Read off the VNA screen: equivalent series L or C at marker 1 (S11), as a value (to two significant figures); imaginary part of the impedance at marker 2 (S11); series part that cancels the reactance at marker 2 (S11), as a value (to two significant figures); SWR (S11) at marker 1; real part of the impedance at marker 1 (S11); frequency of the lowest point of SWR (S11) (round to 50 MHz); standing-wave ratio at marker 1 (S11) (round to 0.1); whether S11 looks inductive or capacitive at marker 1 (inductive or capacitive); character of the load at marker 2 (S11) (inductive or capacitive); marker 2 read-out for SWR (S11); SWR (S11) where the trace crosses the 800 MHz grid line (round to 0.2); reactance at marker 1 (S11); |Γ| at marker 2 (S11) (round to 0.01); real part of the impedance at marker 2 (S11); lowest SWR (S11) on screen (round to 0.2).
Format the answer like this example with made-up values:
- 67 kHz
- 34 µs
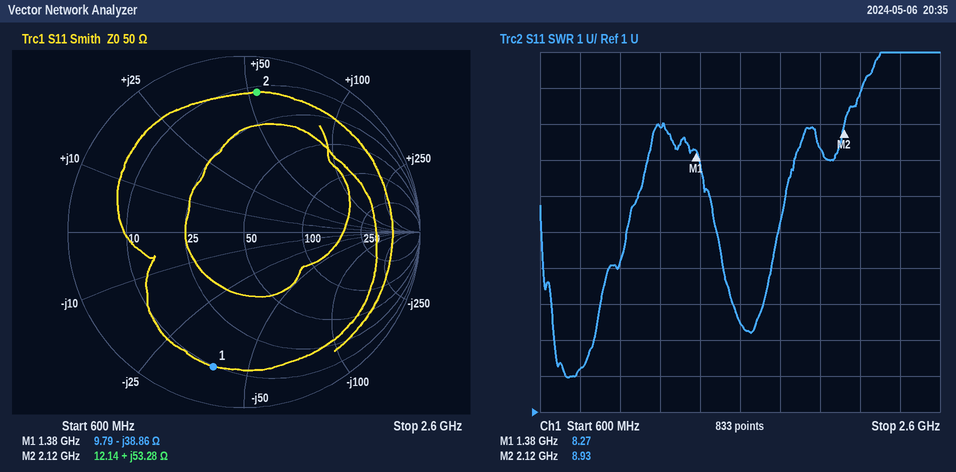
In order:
- 3.0 pF
- +53.28 Ω
- 1.4 pF
- 8.27
- 9.79 Ω
- 750 MHz
- 8.3
- capacitive
- inductive
- 8.93
- 2.2
- -38.86 Ω
- 0.80
- 12.14 Ω
- 2.0
